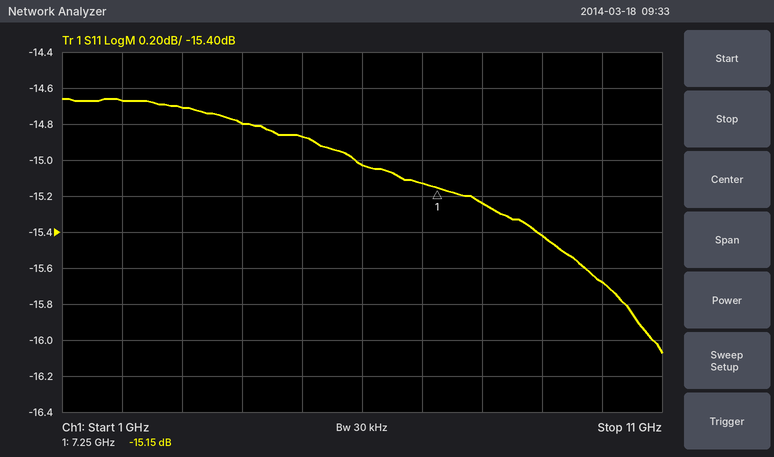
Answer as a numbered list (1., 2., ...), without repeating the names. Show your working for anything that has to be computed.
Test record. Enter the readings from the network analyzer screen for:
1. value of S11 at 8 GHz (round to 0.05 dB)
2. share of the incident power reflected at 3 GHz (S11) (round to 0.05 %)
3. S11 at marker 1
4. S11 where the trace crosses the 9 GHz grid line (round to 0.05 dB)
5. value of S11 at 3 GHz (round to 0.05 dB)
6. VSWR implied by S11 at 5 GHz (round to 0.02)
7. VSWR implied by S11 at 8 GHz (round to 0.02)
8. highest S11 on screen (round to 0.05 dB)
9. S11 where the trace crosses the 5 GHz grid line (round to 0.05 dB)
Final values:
1. -15.25 dB
2. 10^(-14.7/10) ≈ 3.39 %, so 3.40 % to the nearest 0.05 %
3. -15.15 dB
4. -15.40 dB
5. -14.70 dB
6. |Γ| = 10^(-14.85/20) = 0.1809; VSWR = (1 + 0.1809)/(1 − 0.1809) ≈ 1.44
7. |Γ| = 10^(-15.25/20) = 0.1728; VSWR = (1 + 0.1728)/(1 − 0.1728) ≈ 1.42
8. -14.65 dB
9. -14.85 dB
